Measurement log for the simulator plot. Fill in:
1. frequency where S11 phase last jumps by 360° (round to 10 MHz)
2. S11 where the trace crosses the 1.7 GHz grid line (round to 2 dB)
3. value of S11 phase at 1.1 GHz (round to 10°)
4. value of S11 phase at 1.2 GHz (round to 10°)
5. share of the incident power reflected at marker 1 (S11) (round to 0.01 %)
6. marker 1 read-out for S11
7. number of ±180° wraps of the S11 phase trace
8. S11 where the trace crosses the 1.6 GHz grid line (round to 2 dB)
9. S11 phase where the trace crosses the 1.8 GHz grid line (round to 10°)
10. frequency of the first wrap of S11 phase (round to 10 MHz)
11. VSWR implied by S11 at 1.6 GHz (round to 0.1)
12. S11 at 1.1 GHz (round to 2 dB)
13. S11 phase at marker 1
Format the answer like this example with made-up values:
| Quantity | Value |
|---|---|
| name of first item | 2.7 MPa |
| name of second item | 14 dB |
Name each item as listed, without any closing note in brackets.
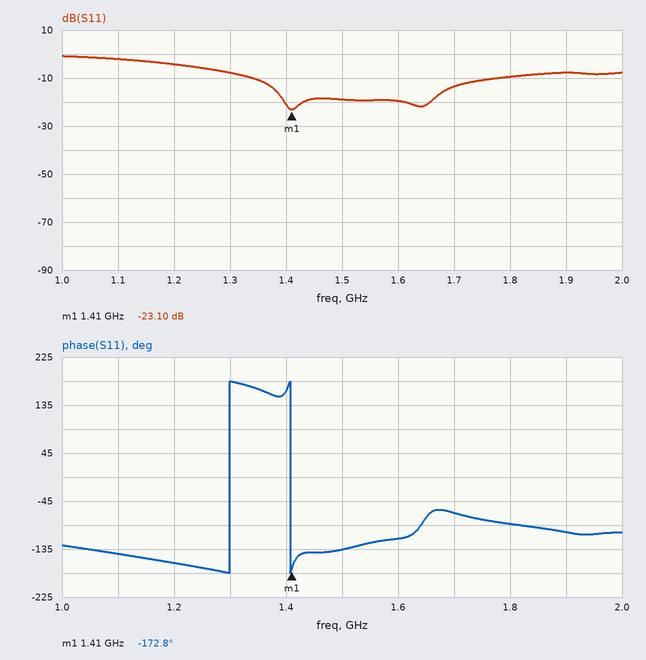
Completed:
| Quantity | Value |
|---|---|
| frequency where S11 phase last jumps by 360° | 1.41 GHz |
| S11 where the trace crosses the 1.7 GHz grid line | -14 dB |
| value of S11 phase at 1.1 GHz | -140° |
| value of S11 phase at 1.2 GHz | -160° |
| share of the incident power reflected at marker 1 (S11) | 0.49 % |
| marker 1 read-out for S11 | -23.10 dB |
| number of ±180° wraps of the S11 phase trace | 2 |
| S11 where the trace crosses the 1.6 GHz grid line | -20 dB |
| S11 phase where the trace crosses the 1.8 GHz grid line | -90° |
| frequency of the first wrap of S11 phase | 1.30 GHz |
| VSWR implied by S11 at 1.6 GHz | 1.2 |
| S11 at 1.1 GHz | -2 dB |
| S11 phase at marker 1 | -172.8° |
